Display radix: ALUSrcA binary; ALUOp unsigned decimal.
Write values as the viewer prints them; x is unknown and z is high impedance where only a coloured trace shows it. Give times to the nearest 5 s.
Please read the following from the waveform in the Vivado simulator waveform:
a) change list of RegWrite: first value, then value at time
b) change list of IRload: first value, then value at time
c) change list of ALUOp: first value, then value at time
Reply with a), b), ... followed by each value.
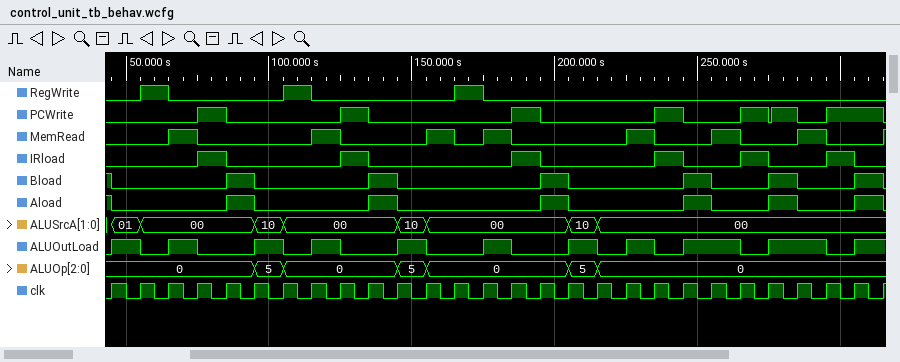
a) 0, 1 at 55 s, 0 at 65 s, 1 at 105 s, 0 at 115 s, 1 at 165 s, 0 at 175 s
b) 0, 1 at 75 s, 0 at 85 s, 1 at 125 s, 0 at 135 s, 1 at 185 s, 0 at 195 s, 1 at 235 s, 0 at 245 s, 1 at 265 s, 0 at 275 s, 1 at 295 s, 0 at 305 s
c) 0, 5 at 95 s, 0 at 105 s, 5 at 145 s, 0 at 155 s, 5 at 205 s, 0 at 215 s
